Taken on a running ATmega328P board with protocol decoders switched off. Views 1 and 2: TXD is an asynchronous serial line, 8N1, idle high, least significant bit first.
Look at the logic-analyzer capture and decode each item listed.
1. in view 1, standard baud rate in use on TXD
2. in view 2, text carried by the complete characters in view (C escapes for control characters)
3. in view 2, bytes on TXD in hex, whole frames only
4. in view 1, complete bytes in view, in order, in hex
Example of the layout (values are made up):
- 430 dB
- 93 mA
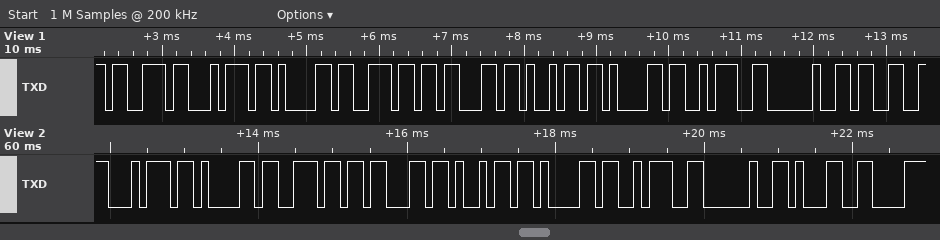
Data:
- 9600 baud
- "tancia: 1"
- 74 61 6E 63 69 61 3A 20 31
- 73 74 61 6E 63 69 61 3A 20 33
